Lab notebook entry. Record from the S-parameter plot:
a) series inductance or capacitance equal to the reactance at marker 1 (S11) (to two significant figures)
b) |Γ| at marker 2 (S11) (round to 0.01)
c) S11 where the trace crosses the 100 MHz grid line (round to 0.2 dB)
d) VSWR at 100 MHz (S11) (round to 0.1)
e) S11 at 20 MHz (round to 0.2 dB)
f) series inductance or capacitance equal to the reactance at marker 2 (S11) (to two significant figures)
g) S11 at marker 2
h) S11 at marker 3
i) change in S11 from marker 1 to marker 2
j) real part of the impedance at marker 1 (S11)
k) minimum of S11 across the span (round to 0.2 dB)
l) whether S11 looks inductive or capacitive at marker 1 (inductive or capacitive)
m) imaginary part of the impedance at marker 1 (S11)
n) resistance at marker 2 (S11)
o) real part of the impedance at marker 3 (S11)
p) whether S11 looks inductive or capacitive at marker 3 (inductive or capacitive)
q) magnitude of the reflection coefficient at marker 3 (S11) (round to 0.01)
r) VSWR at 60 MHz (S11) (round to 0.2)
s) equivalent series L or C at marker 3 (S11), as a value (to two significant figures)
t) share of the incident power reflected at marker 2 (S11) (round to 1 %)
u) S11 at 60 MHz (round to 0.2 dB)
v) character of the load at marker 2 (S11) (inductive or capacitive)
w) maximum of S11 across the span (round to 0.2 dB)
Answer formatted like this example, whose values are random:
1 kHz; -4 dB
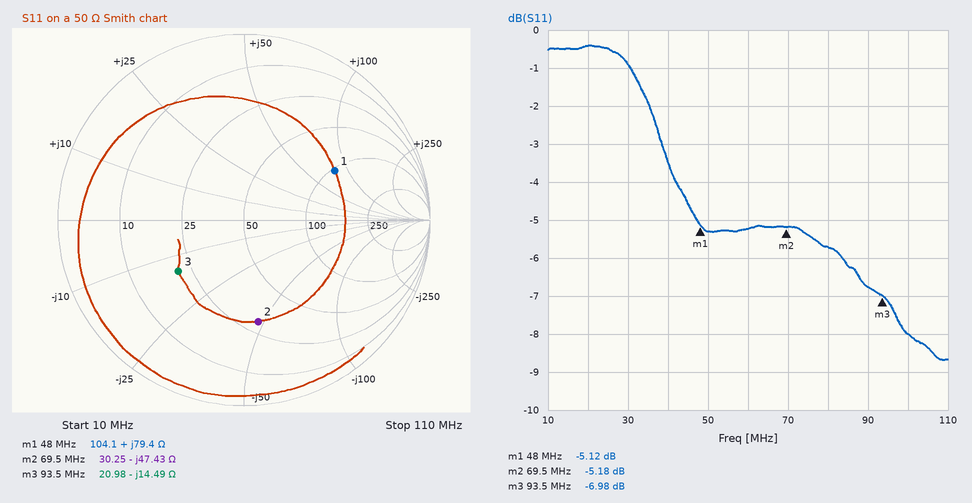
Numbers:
260 nH; 0.55; -8.0 dB; 2.3; -0.4 dB; 48 pF; -5.18 dB; -6.98 dB; -0.06 dB; 104.1 Ω; -8.6 dB; inductive; +79.4 Ω; 30.25 Ω; 20.98 Ω; capacitive; 0.45; 3.4; 120 pF; 30 %; -5.2 dB; capacitive; -0.4 dB
